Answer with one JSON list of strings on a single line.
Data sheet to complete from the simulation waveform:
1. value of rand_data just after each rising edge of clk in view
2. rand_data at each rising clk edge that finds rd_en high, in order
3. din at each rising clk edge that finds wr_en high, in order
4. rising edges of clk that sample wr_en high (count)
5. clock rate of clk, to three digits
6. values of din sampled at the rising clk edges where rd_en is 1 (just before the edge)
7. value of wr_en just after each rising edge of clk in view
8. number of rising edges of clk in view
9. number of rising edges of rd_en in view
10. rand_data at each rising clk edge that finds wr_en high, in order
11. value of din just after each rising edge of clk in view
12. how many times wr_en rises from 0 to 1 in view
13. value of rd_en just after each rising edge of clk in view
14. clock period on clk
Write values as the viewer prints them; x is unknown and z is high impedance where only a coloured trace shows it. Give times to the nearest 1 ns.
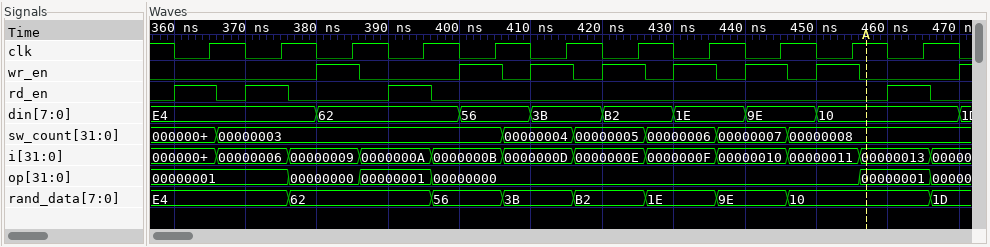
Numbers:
["E4, E4, 62, 62, 56, 3B, B2, 1E, 9E, 10, 10", "E4, E4, 62, 10", "62, 56, 3B, B2, 1E, 9E, 10", "7", "100 MHz", "E4, E4, 62, 10", "0 0 1 0 1 1 1 1 1 1 0", "11", "4", "62, 56, 3B, B2, 1E, 9E, 10", "E4, E4, 62, 62, 56, 3B, B2, 1E, 9E, 10, 10", "8", "1 1 0 1 0 0 0 0 0 0 1", "10 ns"]
